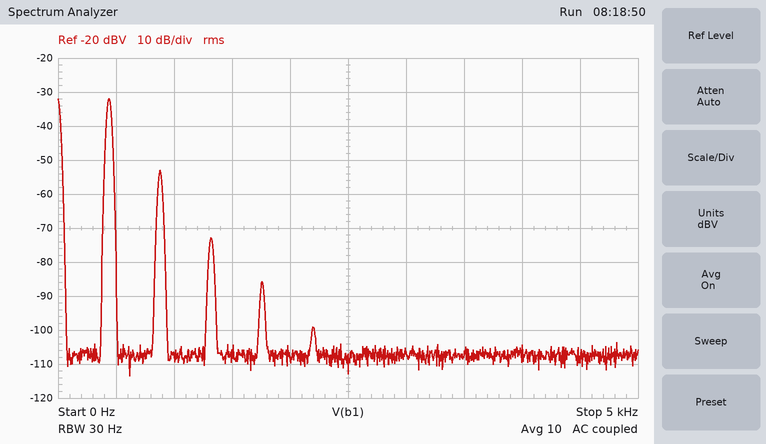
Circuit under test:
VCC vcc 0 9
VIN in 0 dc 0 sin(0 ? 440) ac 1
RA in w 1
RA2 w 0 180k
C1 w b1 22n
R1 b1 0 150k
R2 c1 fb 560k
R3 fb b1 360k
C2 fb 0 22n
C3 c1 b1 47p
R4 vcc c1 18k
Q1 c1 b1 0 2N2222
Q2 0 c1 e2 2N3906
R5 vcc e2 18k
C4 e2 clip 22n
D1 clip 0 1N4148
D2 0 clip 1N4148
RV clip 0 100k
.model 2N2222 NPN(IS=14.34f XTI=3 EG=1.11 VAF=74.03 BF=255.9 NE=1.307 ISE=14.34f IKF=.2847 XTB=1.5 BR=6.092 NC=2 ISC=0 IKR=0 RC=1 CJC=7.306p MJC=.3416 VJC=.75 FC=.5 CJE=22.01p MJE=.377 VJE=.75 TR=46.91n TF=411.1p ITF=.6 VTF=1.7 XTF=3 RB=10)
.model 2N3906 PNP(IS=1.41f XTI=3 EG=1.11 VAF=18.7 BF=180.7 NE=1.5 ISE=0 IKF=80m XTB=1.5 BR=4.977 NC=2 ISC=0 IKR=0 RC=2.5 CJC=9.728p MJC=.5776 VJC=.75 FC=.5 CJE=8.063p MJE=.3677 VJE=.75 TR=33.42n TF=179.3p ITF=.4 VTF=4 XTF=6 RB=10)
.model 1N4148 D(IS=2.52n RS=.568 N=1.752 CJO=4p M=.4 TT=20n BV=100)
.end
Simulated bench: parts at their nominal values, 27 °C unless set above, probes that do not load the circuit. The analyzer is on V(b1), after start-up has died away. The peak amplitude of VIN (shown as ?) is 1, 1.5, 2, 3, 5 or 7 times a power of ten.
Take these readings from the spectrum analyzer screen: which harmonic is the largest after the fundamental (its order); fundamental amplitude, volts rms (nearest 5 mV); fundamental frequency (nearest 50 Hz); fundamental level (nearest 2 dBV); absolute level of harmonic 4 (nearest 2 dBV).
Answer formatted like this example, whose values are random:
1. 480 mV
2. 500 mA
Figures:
1. 2
2. 25 mV
3. 450 Hz
4. -32 dBV
5. -86 dBV
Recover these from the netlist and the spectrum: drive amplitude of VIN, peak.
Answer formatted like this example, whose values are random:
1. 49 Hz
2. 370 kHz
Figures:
1. 50 mV
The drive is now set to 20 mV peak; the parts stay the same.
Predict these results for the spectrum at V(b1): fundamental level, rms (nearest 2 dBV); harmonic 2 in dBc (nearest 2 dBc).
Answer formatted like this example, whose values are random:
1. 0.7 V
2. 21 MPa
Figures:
1. -40 dBV
2. -28 dBc
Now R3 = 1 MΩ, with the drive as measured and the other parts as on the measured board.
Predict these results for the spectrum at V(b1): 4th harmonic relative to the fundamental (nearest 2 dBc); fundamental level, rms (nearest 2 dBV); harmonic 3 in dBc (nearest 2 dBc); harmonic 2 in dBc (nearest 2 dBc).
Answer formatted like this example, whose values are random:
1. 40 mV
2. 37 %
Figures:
1. -60 dBc
2. -30 dBV
3. -42 dBc
4. -26 dBc
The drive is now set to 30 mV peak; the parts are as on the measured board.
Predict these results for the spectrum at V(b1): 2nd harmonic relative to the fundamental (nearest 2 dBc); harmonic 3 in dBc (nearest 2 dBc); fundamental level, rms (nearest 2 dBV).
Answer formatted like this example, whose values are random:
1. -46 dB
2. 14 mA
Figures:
1. -24 dBc
2. -48 dBc
3. -36 dBV
